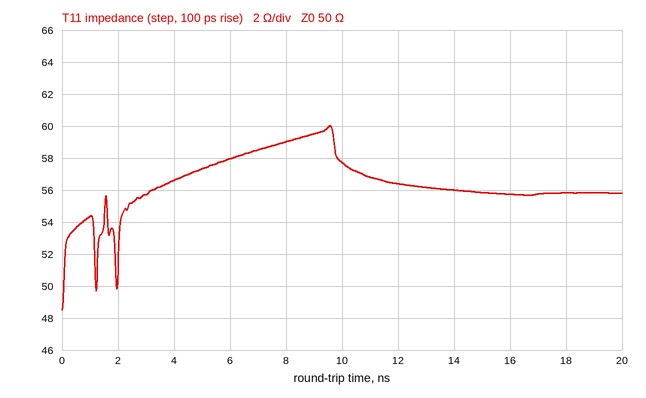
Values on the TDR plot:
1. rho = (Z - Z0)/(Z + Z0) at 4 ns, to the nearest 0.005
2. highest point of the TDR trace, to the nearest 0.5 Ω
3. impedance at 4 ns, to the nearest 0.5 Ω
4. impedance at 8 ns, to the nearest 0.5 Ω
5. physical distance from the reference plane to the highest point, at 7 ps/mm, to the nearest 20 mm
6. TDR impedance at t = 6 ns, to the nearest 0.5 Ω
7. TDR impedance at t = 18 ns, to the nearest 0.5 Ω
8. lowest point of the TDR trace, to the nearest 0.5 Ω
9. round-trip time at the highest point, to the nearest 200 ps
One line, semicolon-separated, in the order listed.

+0.060; 60.0 Ω; 56.5 Ω; 59.0 Ω; 680 mm; 58.0 Ω; 56.0 Ω; 48.5 Ω; 9.6 ns
